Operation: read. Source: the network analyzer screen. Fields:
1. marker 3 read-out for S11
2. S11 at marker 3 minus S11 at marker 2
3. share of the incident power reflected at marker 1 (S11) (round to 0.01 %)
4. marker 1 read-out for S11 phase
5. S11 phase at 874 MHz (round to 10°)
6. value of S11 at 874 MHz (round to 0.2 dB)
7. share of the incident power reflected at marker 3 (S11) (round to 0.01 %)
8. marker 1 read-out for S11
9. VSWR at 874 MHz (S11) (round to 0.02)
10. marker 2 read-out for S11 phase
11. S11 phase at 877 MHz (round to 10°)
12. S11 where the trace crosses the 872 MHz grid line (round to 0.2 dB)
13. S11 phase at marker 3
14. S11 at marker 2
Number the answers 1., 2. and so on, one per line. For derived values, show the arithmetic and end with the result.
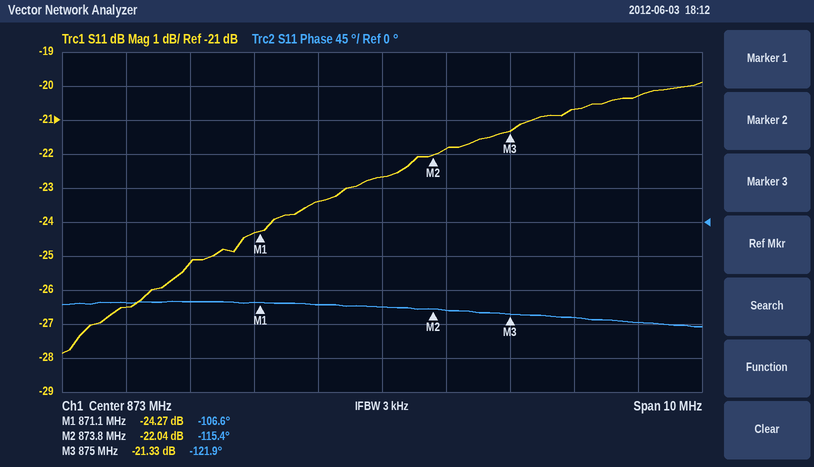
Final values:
1. -21.33 dB
2. -21.33 − (-22.04) = 0.71 dB
3. 10^(-24.27/10) ≈ 0.37 %
4. -106.6°
5. -120°
6. -21.8 dB
7. 10^(-21.33/10) ≈ 0.74 %
8. -24.27 dB
9. |Γ| = 10^(-21.8/20) = 0.0813; VSWR = (1 + 0.0813)/(1 − 0.0813) ≈ 1.18
10. -115.4°
11. -130°
12. -23.4 dB
13. -121.9°
14. -22.04 dB
